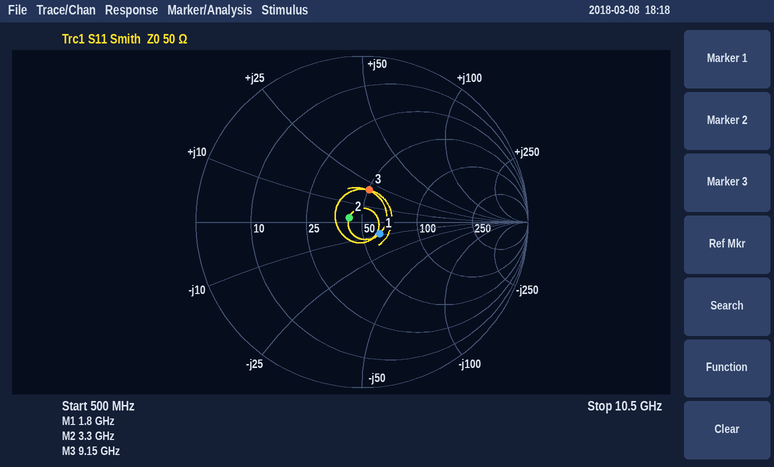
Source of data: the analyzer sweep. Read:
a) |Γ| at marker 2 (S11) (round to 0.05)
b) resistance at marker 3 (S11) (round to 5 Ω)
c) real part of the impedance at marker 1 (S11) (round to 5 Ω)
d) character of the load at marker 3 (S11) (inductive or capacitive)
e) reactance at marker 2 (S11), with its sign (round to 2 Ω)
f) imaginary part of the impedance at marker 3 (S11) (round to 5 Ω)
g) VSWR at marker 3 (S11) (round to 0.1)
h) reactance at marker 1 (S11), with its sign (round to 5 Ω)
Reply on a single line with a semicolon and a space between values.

0.10; 50 Ω; 60 Ω; inductive; +2 Ω; +20 Ω; 1.5; -10 Ω
